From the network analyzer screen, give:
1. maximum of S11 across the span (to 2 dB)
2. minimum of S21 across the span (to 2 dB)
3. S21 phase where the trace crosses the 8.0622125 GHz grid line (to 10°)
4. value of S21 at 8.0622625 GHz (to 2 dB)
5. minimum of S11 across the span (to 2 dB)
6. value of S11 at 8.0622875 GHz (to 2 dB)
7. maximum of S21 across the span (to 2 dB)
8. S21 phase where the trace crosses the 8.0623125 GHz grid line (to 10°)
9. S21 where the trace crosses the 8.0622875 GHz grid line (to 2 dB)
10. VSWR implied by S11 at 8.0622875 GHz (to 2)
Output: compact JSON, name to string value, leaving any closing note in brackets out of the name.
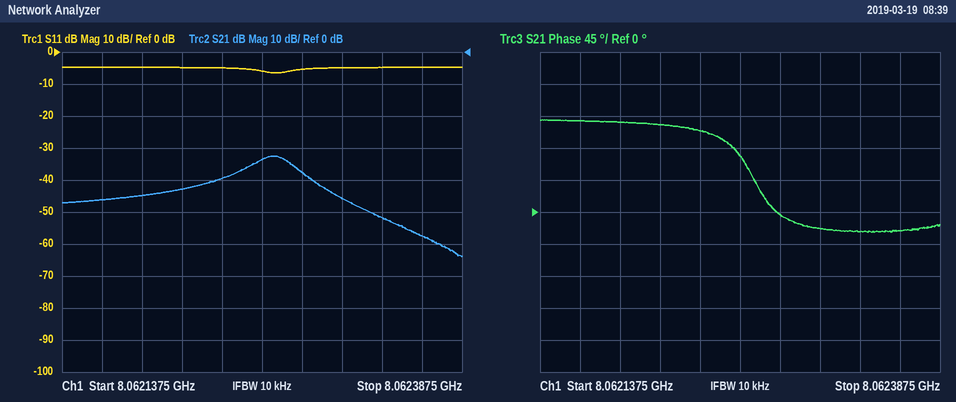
{"maximum of S11 across the span": "-4 dB", "minimum of S21 across the span": "-64 dB", "S21 phase where the trace crosses the 8.0622125 GHz grid line": "120°", "value of S21 at 8.0622625 GHz": "-34 dB", "minimum of S11 across the span": "-6 dB", "value of S11 at 8.0622875 GHz": "-6 dB", "maximum of S21 across the span": "-32 dB", "S21 phase where the trace crosses the 8.0623125 GHz grid line": "-20°", "S21 where the trace crosses the 8.0622875 GHz grid line": "-38 dB", "VSWR implied by S11 at 8.0622875 GHz": "4"}
